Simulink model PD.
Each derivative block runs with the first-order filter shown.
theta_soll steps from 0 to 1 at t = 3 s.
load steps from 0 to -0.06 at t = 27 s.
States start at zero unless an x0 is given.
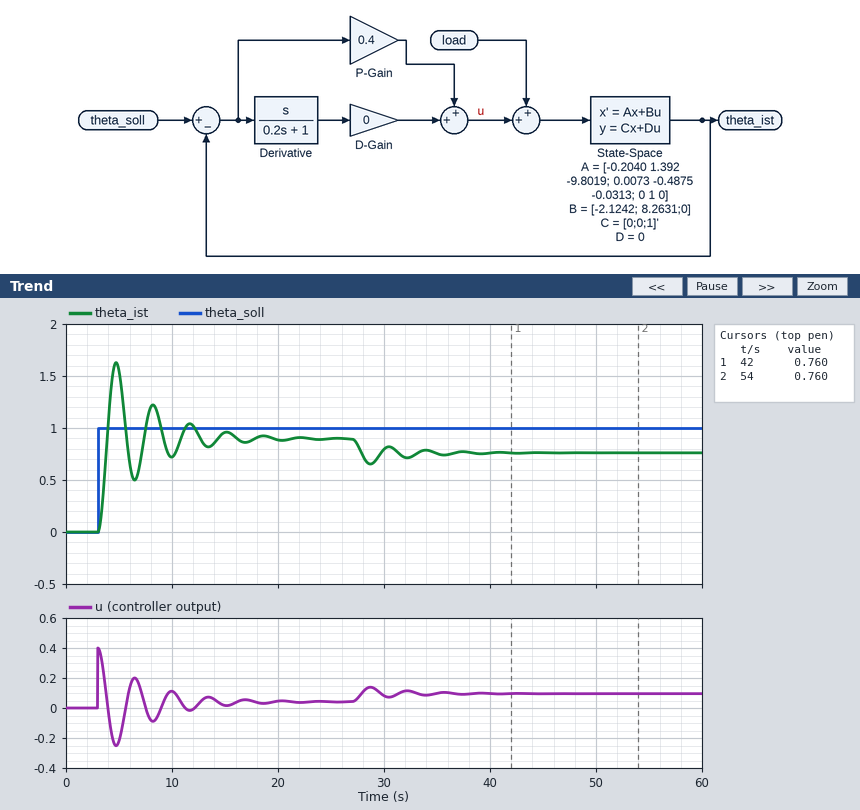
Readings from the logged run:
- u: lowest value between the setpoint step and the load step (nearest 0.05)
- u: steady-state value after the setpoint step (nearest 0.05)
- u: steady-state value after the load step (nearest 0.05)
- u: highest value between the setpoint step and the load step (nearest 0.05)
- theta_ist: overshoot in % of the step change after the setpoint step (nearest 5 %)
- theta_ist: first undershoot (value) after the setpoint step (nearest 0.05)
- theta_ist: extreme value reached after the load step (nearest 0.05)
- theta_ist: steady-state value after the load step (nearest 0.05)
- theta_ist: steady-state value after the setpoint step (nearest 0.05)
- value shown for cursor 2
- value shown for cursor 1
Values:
-0.25
0.05
0.10
0.40
80 %
0.50
0.65
0.75
0.90
0.760
0.760
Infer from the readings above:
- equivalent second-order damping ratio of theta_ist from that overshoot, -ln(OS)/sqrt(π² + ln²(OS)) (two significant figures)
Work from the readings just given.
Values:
0.071
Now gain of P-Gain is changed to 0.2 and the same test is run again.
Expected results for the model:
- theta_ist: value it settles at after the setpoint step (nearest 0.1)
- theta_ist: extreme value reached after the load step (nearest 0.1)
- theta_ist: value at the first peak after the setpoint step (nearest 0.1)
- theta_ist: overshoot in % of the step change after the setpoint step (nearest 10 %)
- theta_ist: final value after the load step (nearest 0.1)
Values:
0.8
0.4
1.5
80 %
0.6
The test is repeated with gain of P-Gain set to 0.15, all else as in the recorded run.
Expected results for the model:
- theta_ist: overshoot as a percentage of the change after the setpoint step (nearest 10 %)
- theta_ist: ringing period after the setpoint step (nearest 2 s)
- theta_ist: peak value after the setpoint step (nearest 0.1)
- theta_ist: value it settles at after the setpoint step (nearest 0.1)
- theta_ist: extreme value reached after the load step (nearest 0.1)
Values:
90 %
6 s
1.4
0.8
0.2
